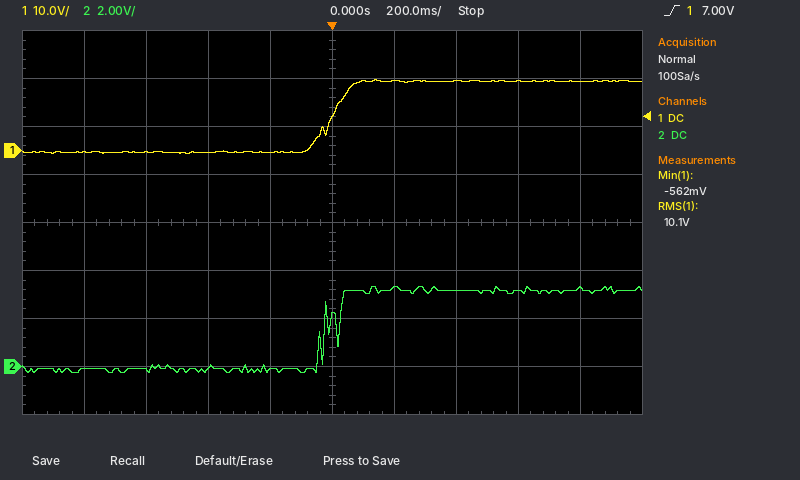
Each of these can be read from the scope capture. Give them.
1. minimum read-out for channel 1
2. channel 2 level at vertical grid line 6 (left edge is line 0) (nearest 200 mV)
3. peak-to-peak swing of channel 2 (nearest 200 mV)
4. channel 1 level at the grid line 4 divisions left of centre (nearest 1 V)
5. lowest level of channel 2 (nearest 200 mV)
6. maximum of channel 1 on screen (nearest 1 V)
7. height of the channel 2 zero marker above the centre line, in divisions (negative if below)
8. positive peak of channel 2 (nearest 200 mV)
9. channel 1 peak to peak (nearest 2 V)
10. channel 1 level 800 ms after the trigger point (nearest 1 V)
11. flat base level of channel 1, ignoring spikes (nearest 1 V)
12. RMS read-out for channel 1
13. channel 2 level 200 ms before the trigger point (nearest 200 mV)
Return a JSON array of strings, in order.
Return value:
["-562 mV", "3.2 V", "3.6 V", "0 V", "-200 mV", "15 V", "-3.0 div", "3.4 V", "16 V", "14 V", "0 V", "10.1 V", "-200 mV"]
